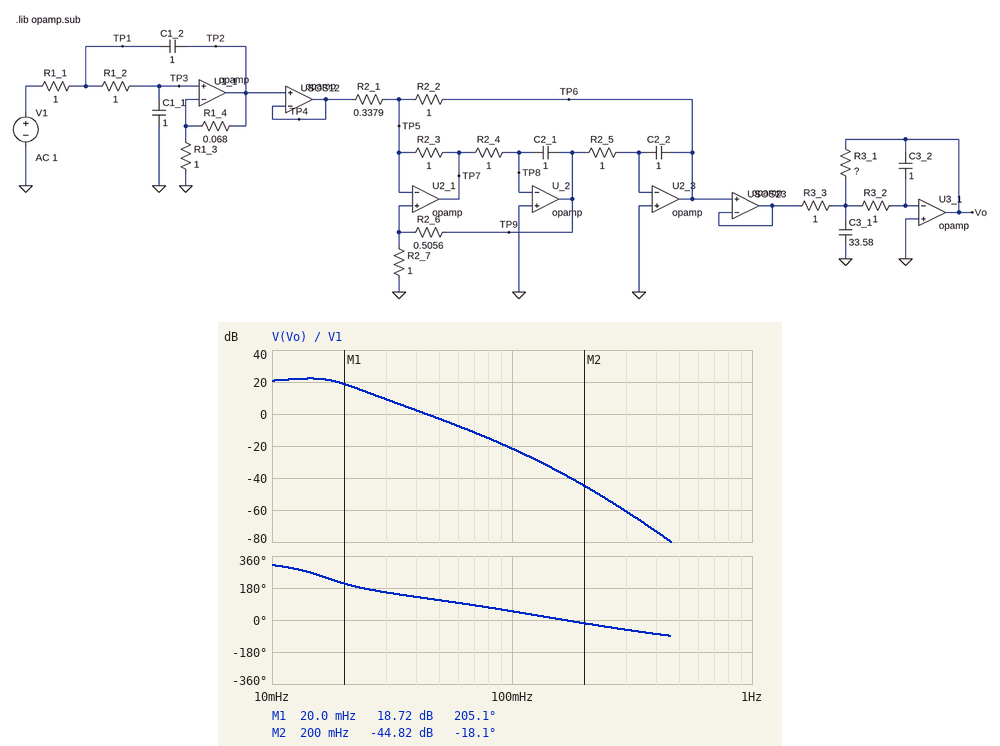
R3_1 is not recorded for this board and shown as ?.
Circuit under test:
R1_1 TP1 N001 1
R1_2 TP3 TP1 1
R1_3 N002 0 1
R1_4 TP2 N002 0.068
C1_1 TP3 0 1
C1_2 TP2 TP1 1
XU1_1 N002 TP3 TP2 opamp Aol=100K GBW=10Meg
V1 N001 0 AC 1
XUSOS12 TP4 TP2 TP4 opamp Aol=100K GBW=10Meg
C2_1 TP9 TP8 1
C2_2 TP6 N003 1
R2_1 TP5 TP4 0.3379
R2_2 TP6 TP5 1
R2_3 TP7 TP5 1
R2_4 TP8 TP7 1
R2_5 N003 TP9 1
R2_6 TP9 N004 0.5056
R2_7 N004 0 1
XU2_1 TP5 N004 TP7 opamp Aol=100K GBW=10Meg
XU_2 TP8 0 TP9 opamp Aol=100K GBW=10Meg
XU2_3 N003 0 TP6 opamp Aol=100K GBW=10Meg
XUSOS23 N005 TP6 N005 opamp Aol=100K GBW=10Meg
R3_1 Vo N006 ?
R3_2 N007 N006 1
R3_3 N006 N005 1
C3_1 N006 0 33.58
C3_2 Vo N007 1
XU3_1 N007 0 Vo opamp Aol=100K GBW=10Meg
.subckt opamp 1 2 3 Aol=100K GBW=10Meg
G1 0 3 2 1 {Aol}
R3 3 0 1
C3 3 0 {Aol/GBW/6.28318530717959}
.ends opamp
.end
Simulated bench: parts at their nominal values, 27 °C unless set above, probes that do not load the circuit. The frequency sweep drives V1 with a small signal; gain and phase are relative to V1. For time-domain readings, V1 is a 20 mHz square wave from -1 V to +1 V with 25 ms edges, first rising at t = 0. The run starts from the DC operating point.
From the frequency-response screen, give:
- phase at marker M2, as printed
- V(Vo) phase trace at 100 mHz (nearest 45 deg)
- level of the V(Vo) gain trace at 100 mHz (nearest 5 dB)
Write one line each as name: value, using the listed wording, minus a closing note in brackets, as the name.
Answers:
phase at marker M2, as printed: -18.1 deg
V(Vo) phase trace at 100 mHz: 45 deg
level of the V(Vo) gain trace at 100 mHz: -20 dB
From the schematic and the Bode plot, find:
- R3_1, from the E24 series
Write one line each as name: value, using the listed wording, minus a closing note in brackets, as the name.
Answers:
R3_1, from the E24 series: 2.7 Ω
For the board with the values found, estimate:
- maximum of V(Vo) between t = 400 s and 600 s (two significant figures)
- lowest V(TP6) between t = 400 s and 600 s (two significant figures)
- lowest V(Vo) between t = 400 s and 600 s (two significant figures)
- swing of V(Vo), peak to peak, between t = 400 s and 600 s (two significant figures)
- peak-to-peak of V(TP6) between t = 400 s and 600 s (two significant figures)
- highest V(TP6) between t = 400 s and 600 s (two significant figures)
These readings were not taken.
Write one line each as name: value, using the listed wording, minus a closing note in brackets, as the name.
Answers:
maximum of V(Vo) between t = 400 s and 600 s: 11 V
lowest V(TP6) between t = 400 s and 600 s: -3.2 V
lowest V(Vo) between t = 400 s and 600 s: -11 V
swing of V(Vo), peak to peak, between t = 400 s and 600 s: 22 V
peak-to-peak of V(TP6) between t = 400 s and 600 s: 6.3 V
highest V(TP6) between t = 400 s and 600 s: 3.2 V
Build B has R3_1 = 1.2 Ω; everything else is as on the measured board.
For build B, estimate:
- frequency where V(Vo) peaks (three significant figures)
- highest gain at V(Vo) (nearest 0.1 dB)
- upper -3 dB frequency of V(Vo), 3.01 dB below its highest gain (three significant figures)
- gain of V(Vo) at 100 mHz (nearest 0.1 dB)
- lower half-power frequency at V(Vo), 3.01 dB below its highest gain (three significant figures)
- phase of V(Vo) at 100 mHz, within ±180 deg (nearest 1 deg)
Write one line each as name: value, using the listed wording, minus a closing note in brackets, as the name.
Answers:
frequency where V(Vo) peaks: 22.8 mHz
highest gain at V(Vo): 16.4 dB
upper -3 dB frequency of V(Vo), 3.01 dB below its highest gain: 28.8 mHz
gain of V(Vo) at 100 mHz: -21.3 dB
lower half-power frequency at V(Vo), 3.01 dB below its highest gain: 13.0 mHz
phase of V(Vo) at 100 mHz, within ±180 deg: 51 deg
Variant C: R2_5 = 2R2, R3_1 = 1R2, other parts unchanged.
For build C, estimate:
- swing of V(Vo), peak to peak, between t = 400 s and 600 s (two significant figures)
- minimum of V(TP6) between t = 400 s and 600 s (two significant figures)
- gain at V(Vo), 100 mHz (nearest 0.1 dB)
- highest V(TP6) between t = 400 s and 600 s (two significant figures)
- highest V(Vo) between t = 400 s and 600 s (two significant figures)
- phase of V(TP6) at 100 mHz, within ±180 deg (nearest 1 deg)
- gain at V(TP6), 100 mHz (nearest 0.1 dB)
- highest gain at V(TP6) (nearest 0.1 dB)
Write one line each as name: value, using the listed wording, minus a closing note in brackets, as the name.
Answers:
swing of V(Vo), peak to peak, between t = 400 s and 600 s: 13 V
minimum of V(TP6) between t = 400 s and 600 s: -2.9 V
gain at V(Vo), 100 mHz: -27.8 dB
highest V(TP6) between t = 400 s and 600 s: 2.9 V
highest V(Vo) between t = 400 s and 600 s: 6.3 V
phase of V(TP6) at 100 mHz, within ±180 deg: 28 deg
gain at V(TP6), 100 mHz: -5.8 dB
highest gain at V(TP6): 10.0 dB
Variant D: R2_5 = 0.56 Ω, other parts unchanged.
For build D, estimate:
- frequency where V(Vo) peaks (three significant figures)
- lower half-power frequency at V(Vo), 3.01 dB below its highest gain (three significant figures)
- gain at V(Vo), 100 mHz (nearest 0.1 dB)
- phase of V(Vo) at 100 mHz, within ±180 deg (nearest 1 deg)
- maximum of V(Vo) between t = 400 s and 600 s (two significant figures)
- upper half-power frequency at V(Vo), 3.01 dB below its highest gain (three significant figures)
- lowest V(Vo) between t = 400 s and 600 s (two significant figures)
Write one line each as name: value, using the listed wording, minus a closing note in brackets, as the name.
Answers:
frequency where V(Vo) peaks: 14.6 mHz
lower half-power frequency at V(Vo), 3.01 dB below its highest gain: 5.86 mHz
gain at V(Vo), 100 mHz: -17.8 dB
phase of V(Vo) at 100 mHz, within ±180 deg: 67 deg
maximum of V(Vo) between t = 400 s and 600 s: 12 V
upper half-power frequency at V(Vo), 3.01 dB below its highest gain: 19.7 mHz
lowest V(Vo) between t = 400 s and 600 s: -12 V
